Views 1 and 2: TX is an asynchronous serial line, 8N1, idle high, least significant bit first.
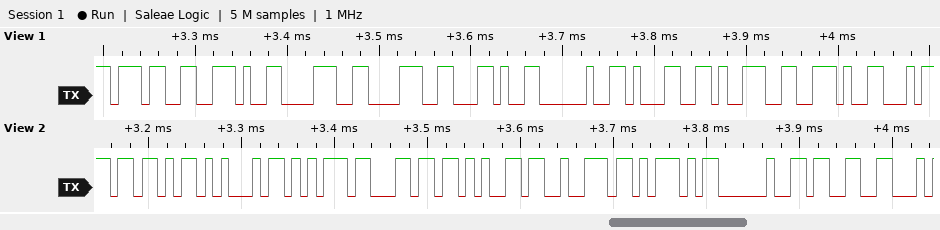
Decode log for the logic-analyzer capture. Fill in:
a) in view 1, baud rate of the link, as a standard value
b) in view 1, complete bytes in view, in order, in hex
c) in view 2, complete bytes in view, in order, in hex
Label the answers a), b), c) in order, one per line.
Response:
a) 115200 baud
b) 37 2E 38 38 2C 20 31 39 2E
c) 5B 45 75 6C 65 72 5D 20 33
